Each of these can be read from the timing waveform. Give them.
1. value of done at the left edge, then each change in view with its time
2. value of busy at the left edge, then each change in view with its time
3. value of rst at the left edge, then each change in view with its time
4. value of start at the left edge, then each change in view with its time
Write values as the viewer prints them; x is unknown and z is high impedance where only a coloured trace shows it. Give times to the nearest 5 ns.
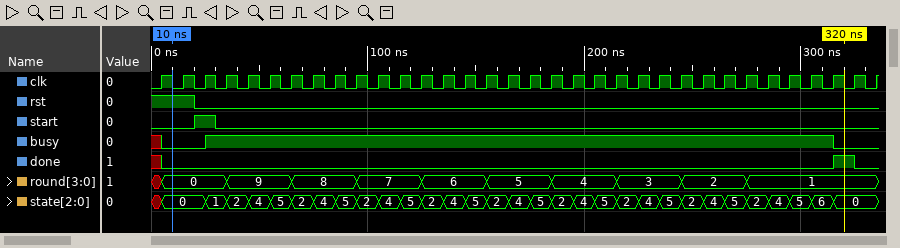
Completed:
x, 0 at 5 ns, 1 at 315 ns, 0 at 325 ns
x, 0 at 5 ns, 1 at 25 ns, 0 at 315 ns
1, 0 at 20 ns
0, 1 at 20 ns, 0 at 30 ns
